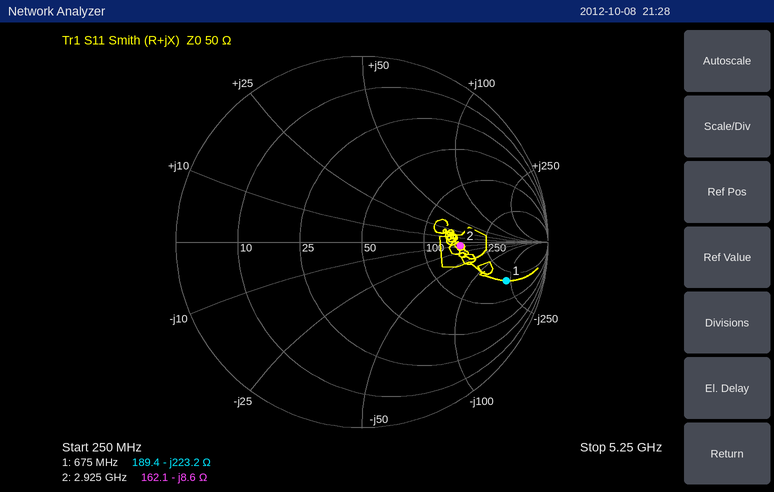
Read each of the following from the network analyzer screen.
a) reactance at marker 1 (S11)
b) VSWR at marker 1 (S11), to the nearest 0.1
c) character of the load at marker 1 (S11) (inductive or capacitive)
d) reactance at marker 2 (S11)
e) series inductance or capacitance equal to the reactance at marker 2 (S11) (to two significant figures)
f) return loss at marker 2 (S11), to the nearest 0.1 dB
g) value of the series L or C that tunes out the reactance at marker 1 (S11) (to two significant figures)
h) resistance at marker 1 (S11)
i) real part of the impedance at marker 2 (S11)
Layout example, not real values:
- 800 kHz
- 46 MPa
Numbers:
- -223.2 Ω
- 9.2
- capacitive
- -8.6 Ω
- 6.3 pF
- 5.5 dB
- 53 nH
- 189.4 Ω
- 162.1 Ω
